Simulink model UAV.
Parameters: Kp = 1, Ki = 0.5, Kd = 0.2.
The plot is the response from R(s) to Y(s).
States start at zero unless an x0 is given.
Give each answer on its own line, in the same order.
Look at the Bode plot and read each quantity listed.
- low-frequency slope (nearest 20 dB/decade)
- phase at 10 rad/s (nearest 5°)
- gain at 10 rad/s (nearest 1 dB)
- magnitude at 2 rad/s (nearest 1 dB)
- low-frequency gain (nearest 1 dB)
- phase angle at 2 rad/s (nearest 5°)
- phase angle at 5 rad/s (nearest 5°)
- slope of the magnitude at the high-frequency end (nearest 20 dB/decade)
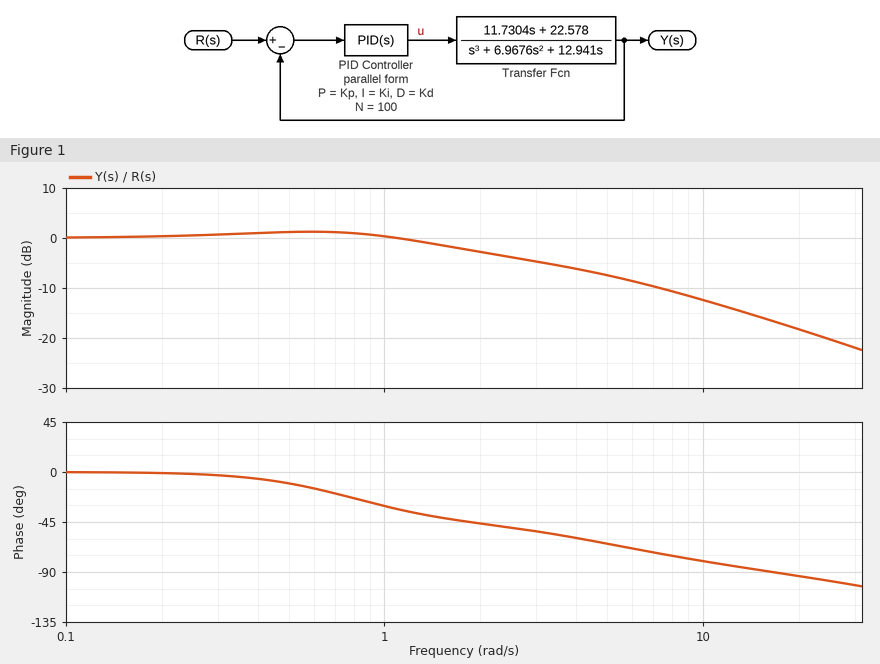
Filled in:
0 dB/decade
-80°
-12 dB
-3 dB
0 dB
-45°
-65°
-20 dB/decade
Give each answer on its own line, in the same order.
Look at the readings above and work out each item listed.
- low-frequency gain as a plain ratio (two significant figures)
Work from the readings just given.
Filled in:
1.0
